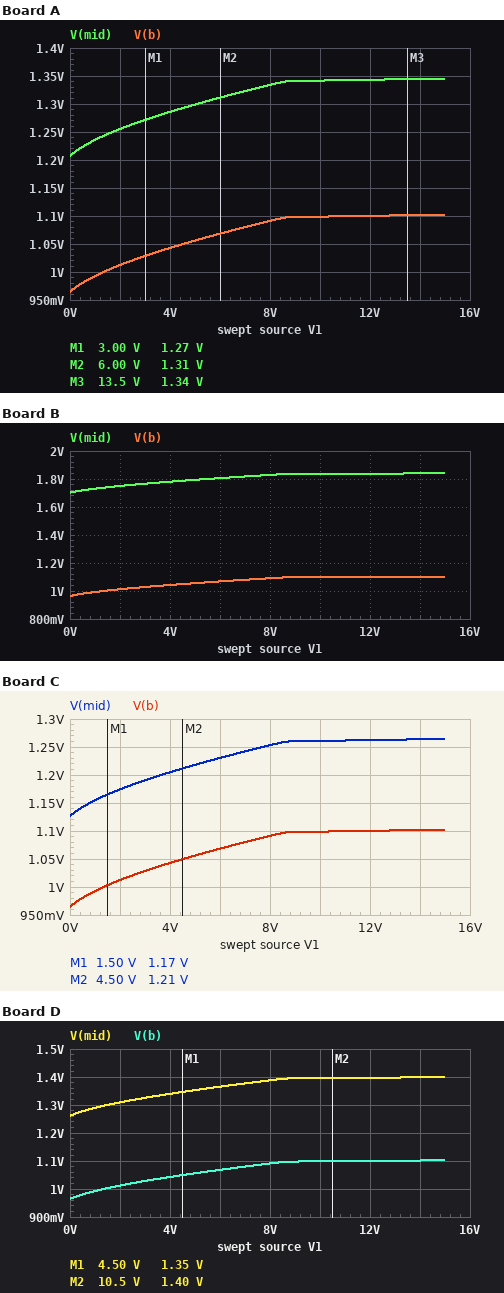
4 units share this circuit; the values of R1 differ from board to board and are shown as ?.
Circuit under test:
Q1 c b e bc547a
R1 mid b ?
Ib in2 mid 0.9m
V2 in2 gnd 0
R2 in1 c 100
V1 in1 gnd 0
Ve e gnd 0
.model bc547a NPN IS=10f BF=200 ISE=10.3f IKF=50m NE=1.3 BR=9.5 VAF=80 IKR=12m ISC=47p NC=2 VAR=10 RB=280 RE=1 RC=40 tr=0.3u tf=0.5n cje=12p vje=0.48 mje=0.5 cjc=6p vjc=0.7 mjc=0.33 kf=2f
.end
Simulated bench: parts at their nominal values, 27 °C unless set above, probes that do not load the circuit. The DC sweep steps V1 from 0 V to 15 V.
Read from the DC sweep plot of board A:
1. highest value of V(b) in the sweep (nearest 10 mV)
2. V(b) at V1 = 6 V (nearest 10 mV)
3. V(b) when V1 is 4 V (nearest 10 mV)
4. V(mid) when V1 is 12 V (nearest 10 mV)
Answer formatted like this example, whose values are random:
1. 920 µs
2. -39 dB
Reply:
1. 1.10 V
2. 1.07 V
3. 1.04 V
4. 1.34 V
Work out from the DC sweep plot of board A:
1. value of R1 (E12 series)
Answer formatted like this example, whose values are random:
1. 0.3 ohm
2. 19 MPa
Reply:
1. 270 Ω
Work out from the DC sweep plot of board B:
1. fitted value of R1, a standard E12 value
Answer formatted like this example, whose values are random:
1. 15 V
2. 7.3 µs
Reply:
1. 820 Ω
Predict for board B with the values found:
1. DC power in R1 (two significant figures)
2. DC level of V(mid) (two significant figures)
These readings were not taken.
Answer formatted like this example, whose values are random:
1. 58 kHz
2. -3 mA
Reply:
1. 660 µW
2. 1.7 V
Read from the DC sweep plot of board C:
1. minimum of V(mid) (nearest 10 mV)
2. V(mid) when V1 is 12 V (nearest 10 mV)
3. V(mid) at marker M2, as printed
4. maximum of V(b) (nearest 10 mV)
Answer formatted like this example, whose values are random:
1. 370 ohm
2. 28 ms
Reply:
1. 1.13 V
2. 1.26 V
3. 1.21 V
4. 1.10 V
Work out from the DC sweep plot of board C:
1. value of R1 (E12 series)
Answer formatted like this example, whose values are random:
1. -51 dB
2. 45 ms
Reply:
1. 180 Ω
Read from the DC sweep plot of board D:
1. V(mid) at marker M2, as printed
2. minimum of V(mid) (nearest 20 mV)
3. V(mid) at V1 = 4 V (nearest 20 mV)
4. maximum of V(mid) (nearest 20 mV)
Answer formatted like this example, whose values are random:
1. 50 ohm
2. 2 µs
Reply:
1. 1.40 V
2. 1.26 V
3. 1.34 V
4. 1.40 V
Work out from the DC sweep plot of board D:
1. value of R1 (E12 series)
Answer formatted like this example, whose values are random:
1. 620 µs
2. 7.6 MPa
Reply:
1. 330 Ω
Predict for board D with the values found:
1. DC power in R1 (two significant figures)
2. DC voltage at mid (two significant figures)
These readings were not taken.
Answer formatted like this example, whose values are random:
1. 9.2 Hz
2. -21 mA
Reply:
1. 270 µW
2. 1.3 V
